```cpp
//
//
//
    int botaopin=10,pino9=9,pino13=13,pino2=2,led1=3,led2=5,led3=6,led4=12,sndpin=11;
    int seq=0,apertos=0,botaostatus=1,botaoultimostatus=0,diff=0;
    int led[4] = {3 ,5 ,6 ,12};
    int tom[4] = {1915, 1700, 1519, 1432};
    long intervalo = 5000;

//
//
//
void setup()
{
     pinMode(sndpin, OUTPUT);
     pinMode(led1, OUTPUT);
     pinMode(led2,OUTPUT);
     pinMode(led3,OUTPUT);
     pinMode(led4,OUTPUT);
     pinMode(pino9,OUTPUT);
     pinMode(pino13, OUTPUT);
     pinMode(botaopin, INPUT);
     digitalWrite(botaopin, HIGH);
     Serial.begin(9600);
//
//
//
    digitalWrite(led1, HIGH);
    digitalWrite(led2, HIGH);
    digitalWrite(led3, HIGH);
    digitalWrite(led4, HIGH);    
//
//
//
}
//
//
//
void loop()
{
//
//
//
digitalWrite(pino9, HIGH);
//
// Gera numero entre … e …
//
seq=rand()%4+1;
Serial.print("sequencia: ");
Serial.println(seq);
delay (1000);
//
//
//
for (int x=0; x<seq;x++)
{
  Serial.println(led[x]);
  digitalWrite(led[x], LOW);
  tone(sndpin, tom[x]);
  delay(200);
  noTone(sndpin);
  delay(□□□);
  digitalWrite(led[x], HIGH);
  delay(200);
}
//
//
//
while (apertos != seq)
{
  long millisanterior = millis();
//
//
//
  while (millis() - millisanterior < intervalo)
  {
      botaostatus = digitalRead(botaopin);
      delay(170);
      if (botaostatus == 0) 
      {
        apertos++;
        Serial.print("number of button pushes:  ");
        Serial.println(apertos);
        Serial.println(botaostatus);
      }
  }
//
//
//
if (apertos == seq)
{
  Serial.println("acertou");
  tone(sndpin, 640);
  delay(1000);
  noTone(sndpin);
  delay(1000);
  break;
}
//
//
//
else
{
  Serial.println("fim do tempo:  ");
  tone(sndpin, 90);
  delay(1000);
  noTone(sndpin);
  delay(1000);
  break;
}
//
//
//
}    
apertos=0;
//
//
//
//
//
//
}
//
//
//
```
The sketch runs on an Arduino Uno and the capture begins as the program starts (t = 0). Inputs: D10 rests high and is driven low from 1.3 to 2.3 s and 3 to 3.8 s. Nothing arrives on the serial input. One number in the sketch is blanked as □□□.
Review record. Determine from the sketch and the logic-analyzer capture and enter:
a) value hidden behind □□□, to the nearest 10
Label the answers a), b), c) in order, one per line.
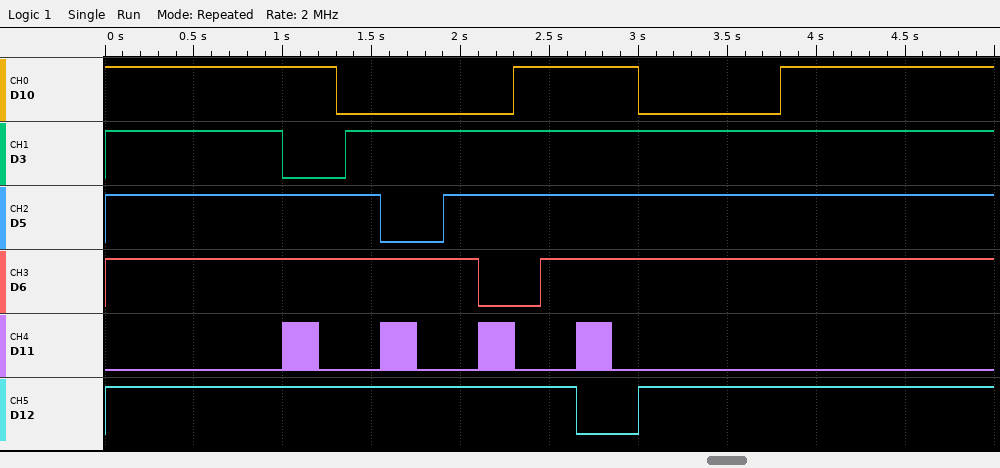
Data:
a) 150
